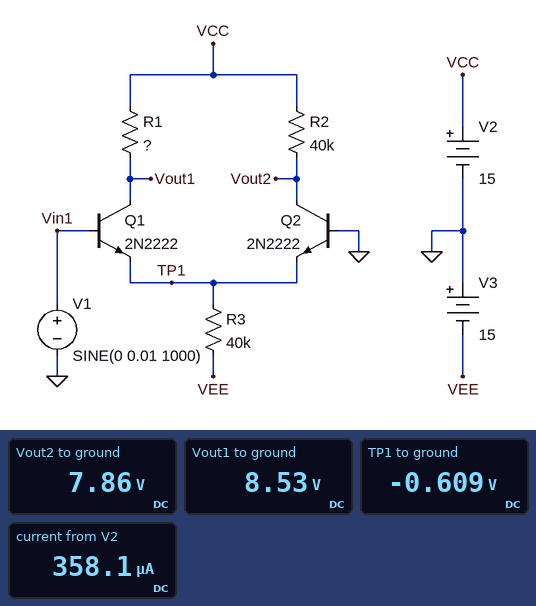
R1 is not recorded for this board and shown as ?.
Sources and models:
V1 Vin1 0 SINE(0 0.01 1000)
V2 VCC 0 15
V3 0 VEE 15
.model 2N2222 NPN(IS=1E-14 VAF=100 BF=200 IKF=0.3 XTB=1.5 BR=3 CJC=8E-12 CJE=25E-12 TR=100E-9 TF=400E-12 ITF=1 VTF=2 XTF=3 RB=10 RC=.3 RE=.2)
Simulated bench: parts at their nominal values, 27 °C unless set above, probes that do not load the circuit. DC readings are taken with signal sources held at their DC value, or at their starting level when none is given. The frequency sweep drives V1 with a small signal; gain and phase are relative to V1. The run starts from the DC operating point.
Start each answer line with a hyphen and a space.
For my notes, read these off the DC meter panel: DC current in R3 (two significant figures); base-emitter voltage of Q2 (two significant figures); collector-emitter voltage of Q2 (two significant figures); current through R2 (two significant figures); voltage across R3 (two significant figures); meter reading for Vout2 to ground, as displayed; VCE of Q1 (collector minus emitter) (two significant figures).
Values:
- 360 µA
- 610 mV
- 8.5 V
- 180 µA
- 14 V
- 7.86 V
- 9.1 V
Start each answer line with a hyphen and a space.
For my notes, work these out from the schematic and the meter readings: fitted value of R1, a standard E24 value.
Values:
- 36 kΩ
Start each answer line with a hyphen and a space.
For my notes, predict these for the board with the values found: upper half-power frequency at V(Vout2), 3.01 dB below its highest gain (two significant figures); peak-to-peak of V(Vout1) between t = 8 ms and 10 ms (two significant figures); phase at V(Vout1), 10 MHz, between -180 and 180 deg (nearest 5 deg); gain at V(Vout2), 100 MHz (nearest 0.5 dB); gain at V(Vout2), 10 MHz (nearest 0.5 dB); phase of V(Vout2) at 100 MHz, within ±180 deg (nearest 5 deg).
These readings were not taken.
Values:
- 1.1 MHz
- 2.3 V
- 90 deg
- 2.0 dB
- 23.0 dB
- -100 deg
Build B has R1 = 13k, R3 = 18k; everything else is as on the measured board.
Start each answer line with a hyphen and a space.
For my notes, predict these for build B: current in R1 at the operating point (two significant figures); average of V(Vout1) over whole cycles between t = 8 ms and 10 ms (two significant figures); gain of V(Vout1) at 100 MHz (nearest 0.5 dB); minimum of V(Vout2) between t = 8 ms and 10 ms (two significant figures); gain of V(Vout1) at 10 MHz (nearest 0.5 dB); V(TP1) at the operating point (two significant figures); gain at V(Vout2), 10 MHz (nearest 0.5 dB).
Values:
- 420 µA
- 9.5 V
- 10.5 dB
- -590 mV
- 29.5 dB
- -630 mV
- 21.5 dB
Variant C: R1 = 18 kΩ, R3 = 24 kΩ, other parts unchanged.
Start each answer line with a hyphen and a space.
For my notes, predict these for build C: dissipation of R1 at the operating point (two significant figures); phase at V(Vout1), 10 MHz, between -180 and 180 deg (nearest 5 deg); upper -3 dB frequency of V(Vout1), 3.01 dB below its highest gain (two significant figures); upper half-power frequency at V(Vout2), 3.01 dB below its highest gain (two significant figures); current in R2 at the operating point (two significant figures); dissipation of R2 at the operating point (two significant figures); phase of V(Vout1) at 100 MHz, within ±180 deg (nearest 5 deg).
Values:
- 1.7 mW
- 100 deg
- 2.5 MHz
- 870 kHz
- 290 µA
- 3.4 mW
- 60 deg
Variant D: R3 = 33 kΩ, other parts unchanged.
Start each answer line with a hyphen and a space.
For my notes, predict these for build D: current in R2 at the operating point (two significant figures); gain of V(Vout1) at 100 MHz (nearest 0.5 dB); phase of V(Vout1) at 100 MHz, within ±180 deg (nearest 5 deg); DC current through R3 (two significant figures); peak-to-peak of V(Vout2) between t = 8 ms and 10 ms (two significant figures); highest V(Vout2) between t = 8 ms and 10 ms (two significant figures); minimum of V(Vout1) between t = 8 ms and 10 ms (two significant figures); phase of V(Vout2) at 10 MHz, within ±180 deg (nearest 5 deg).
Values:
- 220 µA
- 6.0 dB
- 50 deg
- 440 µA
- 3.1 V
- 7.9 V
- 5.8 V
- -85 deg
